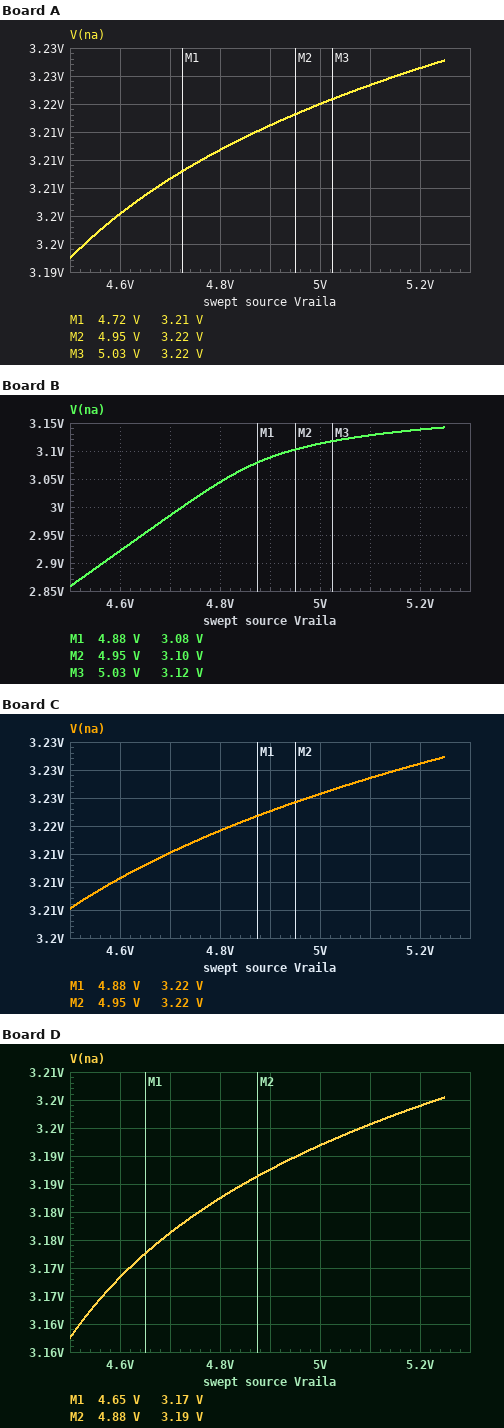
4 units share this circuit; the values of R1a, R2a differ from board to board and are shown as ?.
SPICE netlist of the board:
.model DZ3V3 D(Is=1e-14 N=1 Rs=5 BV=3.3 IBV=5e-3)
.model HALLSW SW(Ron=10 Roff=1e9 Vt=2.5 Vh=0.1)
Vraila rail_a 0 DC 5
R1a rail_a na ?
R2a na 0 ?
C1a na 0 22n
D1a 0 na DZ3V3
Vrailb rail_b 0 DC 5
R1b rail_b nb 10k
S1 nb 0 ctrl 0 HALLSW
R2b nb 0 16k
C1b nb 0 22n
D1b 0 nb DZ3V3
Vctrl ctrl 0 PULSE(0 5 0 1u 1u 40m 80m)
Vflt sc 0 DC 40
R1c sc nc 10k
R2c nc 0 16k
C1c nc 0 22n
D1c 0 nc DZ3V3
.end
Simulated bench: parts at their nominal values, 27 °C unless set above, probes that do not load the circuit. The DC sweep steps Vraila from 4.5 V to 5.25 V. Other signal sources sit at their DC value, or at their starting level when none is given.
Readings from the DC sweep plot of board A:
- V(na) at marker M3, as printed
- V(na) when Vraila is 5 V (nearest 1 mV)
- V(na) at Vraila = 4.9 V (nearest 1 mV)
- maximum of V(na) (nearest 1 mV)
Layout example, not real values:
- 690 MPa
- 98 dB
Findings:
- 3.22 V
- 3.220 V
- 3.216 V
- 3.228 V
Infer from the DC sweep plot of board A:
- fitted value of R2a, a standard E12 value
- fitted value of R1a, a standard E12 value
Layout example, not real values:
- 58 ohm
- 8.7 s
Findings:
- 10 kΩ
- 3.3 kΩ
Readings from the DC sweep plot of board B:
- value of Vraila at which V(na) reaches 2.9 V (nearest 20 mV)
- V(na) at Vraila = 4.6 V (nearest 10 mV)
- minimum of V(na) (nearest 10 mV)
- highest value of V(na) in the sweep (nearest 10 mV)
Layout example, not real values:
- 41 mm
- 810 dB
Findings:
- 4.56 V
- 2.92 V
- 2.86 V
- 3.14 V
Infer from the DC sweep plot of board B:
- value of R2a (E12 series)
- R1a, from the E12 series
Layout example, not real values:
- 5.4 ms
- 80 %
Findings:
- 47 kΩ
- 27 kΩ
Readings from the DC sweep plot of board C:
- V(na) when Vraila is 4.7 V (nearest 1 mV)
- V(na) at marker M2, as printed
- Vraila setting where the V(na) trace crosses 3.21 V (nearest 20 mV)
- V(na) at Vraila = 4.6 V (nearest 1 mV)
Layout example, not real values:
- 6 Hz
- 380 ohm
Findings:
- 3.215 V
- 3.22 V
- 4.70 V
- 3.211 V
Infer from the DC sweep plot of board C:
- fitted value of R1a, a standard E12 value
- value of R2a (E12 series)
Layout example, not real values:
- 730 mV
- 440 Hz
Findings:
- 3.3 kΩ
- 12 kΩ
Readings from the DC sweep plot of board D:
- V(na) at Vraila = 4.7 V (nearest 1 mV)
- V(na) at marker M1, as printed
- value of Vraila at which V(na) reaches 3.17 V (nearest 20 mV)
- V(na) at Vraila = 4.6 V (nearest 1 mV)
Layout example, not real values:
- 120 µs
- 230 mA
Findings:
- 3.176 V
- 3.17 V
- 4.56 V
- 3.168 V
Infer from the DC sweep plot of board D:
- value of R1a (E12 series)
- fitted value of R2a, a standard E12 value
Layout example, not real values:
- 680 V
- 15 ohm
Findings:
- 8.2 kΩ
- 22 kΩ
